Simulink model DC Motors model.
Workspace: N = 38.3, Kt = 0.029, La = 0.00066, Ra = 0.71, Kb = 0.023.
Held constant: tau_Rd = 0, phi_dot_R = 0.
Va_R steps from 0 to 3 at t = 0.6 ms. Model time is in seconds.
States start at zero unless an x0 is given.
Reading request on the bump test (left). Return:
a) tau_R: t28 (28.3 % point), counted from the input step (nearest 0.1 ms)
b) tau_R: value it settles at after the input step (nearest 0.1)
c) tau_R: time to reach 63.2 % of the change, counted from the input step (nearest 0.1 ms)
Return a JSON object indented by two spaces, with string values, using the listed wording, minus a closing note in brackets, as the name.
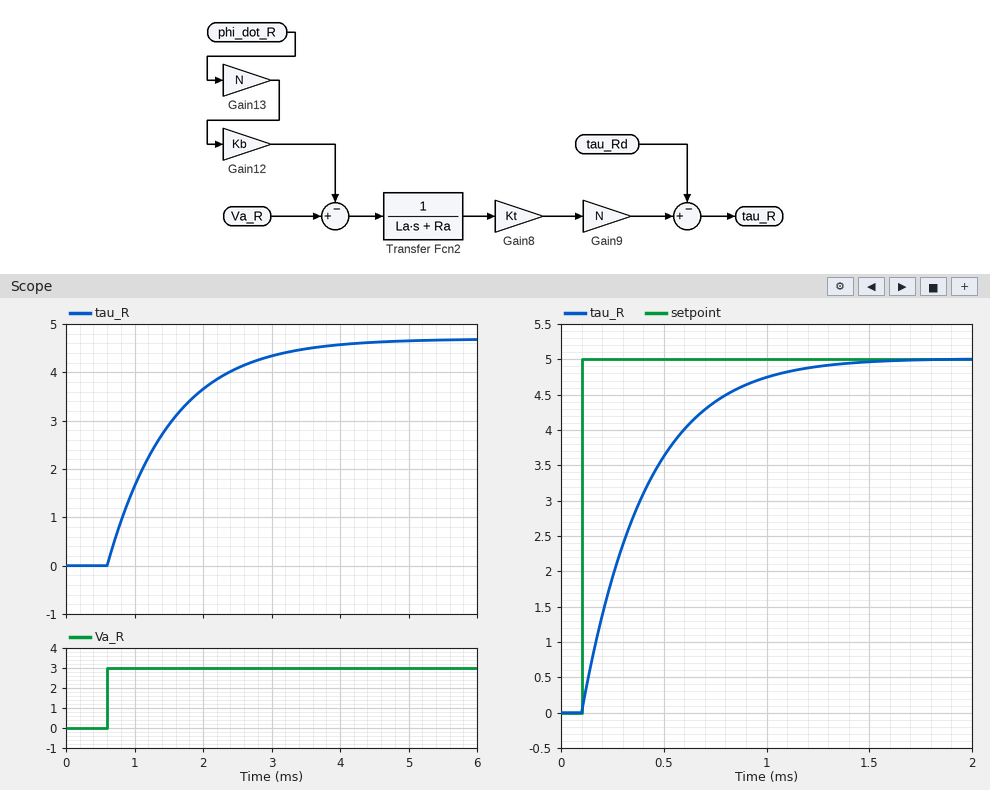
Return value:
{
  "tau_R: t28 (28.3 % point), counted from the input step": "0.3 ms",
  "tau_R: value it settles at after the input step": "4.7",
  "tau_R: time to reach 63.2 % of the change, counted from the input step": "0.9 ms"
}
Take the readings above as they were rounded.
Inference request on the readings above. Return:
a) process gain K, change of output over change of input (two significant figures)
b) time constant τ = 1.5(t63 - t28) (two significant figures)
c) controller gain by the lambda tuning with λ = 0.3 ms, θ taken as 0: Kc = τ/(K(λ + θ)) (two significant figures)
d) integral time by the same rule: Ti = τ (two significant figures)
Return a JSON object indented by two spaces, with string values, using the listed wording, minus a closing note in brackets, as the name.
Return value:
{
  "process gain K, change of output over change of input": "1.6",
  "time constant τ = 1.5(t63 - t28)": "0.90 ms",
  "controller gain by the lambda tuning with λ = 0.3 ms, θ taken as 0: Kc = τ/(K(λ + θ))": "1.9",
  "integral time by the same rule: Ti = τ": "0.90 ms"
}
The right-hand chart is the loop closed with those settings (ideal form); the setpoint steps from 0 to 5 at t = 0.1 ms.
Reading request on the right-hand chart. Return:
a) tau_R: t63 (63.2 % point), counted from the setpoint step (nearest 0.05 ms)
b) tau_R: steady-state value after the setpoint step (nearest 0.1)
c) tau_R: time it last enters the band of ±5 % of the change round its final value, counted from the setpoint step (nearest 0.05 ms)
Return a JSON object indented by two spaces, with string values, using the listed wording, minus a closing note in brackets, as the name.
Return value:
{
  "tau_R: t63 (63.2 % point), counted from the setpoint step": "0.30 ms",
  "tau_R: steady-state value after the setpoint step": "5.0",
  "tau_R: time it last enters the band of ±5 % of the change round its final value, counted from the setpoint step": "0.90 ms"
}
